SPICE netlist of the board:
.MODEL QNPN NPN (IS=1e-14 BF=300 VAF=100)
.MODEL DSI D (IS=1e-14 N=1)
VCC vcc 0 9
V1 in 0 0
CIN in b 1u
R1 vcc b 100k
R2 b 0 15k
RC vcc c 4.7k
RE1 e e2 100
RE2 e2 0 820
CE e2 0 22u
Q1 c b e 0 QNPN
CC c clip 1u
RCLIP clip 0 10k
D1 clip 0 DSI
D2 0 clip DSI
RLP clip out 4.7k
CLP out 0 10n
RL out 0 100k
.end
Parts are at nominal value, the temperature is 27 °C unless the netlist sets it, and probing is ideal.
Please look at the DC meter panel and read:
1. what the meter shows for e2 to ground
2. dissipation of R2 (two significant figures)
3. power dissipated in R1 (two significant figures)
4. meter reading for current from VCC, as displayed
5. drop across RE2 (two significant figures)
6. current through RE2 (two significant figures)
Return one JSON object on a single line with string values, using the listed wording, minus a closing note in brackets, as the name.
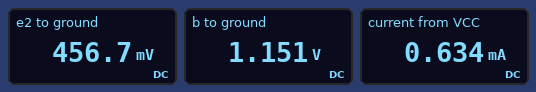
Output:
{"what the meter shows for e2 to ground": "456.7 mV", "dissipation of R2": "88 µW", "power dissipated in R1": "620 µW", "meter reading for current from VCC, as displayed": "0.634 mA", "drop across RE2": "460 mV", "current through RE2": "560 µA"}
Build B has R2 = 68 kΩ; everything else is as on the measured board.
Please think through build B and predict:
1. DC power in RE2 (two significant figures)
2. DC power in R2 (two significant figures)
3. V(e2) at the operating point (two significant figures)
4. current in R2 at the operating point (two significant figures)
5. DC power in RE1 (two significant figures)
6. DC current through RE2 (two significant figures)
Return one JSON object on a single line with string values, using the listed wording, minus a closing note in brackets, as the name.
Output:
{"DC power in RE2": "2.1 mW", "DC power in R2": "68 µW", "V(e2) at the operating point": "1.3 V", "current in R2 at the operating point": "32 µA", "DC power in RE1": "260 µW", "DC current through RE2": "1.6 mA"}
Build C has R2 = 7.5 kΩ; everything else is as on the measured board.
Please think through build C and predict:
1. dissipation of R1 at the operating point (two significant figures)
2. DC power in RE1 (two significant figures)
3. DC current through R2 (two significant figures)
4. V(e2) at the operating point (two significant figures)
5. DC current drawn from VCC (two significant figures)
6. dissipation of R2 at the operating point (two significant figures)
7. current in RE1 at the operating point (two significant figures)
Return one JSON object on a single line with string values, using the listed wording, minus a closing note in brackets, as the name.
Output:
{"dissipation of R1 at the operating point": "700 µW", "DC power in RE1": "290 nW", "DC current through R2": "84 µA", "V(e2) at the operating point": "44 mV", "DC current drawn from VCC": "140 µA", "dissipation of R2 at the operating point": "52 µW", "current in RE1 at the operating point": "54 µA"}
